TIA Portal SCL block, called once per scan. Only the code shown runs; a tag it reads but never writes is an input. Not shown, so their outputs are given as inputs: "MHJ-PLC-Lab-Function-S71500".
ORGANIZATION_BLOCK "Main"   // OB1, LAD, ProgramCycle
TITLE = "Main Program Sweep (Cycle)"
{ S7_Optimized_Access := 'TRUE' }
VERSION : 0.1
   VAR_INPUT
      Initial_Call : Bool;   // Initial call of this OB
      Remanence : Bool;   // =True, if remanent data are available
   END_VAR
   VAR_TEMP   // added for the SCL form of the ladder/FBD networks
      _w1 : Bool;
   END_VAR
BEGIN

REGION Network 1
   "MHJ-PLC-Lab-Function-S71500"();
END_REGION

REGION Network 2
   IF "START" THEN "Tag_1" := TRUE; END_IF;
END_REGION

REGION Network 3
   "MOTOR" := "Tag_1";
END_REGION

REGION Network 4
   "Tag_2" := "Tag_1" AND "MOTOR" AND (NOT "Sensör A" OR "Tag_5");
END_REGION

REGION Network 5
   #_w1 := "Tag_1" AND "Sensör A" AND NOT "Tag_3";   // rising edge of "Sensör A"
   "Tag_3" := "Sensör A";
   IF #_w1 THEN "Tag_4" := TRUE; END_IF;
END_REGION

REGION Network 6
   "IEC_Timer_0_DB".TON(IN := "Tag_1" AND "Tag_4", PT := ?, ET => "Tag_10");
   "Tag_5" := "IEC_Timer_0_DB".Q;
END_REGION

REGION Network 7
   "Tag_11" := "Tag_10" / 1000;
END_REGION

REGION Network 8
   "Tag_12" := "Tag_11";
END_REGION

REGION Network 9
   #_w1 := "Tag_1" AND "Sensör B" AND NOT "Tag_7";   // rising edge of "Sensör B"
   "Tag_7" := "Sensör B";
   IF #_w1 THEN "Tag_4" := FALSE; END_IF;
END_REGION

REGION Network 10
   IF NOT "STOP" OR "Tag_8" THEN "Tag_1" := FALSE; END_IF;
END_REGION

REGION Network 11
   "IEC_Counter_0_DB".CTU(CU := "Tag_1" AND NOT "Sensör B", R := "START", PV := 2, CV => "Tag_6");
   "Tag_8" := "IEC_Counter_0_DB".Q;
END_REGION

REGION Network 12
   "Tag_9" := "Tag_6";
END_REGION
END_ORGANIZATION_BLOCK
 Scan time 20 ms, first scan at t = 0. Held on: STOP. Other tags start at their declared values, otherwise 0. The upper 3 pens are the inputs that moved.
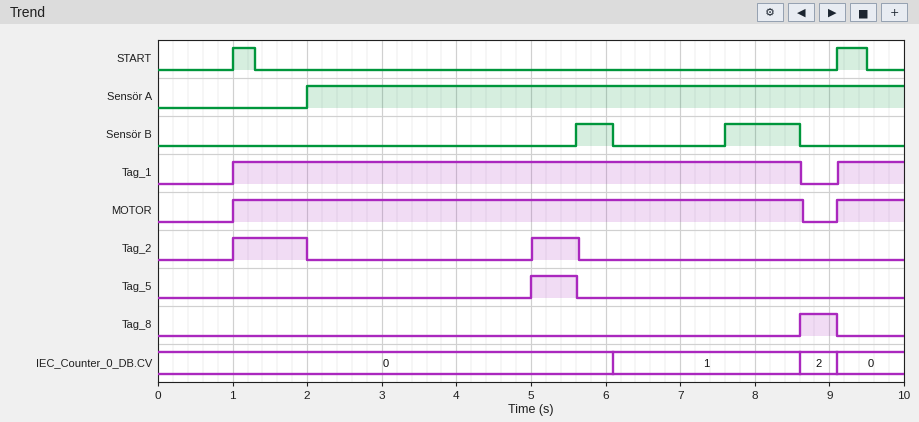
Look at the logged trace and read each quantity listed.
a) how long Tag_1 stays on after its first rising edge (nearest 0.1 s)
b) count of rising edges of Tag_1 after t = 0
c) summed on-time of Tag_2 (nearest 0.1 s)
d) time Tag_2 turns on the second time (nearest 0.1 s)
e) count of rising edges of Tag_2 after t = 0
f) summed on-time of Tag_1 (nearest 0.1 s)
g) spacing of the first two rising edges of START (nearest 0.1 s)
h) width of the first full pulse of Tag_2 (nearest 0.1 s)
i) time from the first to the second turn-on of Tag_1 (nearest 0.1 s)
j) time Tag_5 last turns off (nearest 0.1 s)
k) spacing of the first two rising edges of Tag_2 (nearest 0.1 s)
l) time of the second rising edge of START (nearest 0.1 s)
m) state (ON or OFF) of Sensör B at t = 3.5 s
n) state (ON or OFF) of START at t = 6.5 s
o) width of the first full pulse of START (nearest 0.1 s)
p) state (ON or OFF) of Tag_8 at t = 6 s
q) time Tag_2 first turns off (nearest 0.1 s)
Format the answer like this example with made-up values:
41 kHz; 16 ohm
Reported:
7.6 s; 2; 1.6 s; 5.0 s; 2; 8.5 s; 8.1 s; 1.0 s; 8.1 s; 5.6 s; 4.0 s; 9.1 s; OFF; OFF; 0.3 s; OFF; 2.0 s
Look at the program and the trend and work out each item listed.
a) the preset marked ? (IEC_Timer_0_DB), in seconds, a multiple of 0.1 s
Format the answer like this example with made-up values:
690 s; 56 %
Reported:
3.0 s
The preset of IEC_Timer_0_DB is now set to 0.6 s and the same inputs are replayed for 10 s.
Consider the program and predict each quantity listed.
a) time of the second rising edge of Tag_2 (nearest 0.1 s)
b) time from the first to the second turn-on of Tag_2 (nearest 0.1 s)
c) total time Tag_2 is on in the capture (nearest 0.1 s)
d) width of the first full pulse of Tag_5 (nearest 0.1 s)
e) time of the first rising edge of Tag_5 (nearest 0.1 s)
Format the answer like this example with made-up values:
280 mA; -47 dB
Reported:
2.6 s; 1.6 s; 4.0 s; 3.0 s; 2.6 s
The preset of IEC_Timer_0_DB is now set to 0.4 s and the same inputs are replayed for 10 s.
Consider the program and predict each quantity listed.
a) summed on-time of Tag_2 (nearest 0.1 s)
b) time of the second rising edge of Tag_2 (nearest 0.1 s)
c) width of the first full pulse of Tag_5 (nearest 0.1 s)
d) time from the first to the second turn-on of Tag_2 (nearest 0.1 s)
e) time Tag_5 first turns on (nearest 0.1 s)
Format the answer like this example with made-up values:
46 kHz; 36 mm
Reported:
4.2 s; 2.4 s; 3.2 s; 1.4 s; 2.4 s
